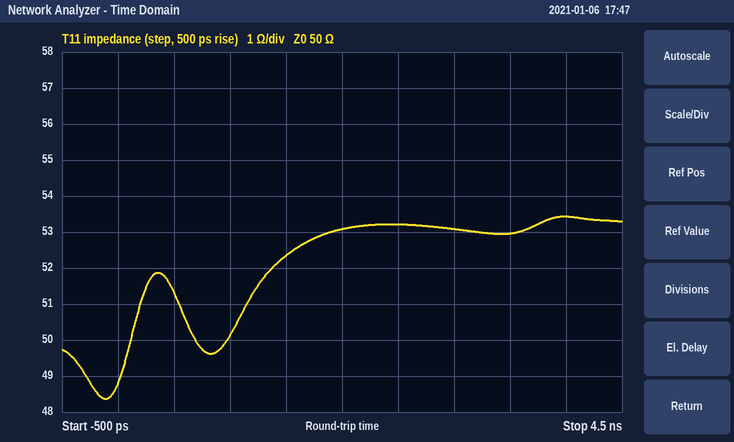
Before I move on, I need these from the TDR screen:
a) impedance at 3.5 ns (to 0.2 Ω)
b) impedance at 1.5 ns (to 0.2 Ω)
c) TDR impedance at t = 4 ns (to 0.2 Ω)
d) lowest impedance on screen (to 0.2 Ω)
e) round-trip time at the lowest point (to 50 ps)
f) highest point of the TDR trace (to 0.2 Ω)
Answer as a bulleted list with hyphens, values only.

- 53.0 Ω
- 52.4 Ω
- 53.4 Ω
- 48.4 Ω
- -100 ps
- 53.4 Ω
